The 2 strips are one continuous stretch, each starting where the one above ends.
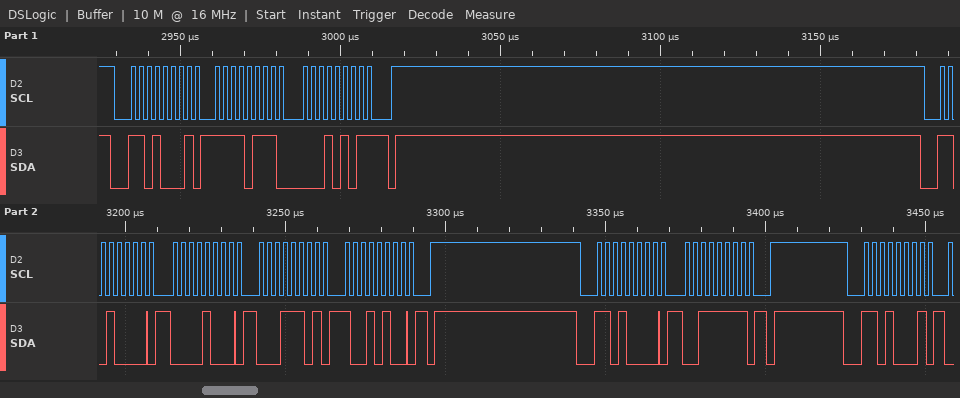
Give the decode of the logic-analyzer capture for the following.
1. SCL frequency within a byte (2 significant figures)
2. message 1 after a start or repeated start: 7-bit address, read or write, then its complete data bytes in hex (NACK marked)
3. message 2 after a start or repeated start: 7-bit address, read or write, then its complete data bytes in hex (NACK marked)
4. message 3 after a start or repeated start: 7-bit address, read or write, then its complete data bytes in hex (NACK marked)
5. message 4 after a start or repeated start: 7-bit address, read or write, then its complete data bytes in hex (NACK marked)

400 kHz
0x68 read: F7 15 NACK
0x68 write: 08 1D 94
0x68 write: 3F
0x68 read
